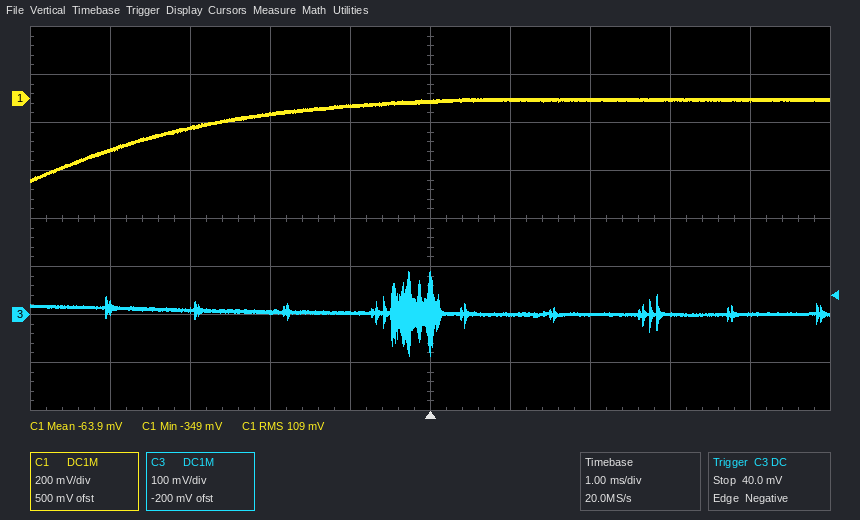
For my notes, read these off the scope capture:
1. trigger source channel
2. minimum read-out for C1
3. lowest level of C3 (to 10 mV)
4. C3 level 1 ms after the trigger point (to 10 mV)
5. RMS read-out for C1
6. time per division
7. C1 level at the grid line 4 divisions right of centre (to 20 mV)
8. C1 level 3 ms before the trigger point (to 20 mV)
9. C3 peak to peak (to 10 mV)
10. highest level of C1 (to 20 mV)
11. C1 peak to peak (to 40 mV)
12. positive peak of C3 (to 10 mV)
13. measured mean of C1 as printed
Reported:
C3
-349 mV
-90 mV
0 mV
109 mV
1 ms
0 mV
-120 mV
180 mV
0 mV
360 mV
90 mV
-63.9 mV
